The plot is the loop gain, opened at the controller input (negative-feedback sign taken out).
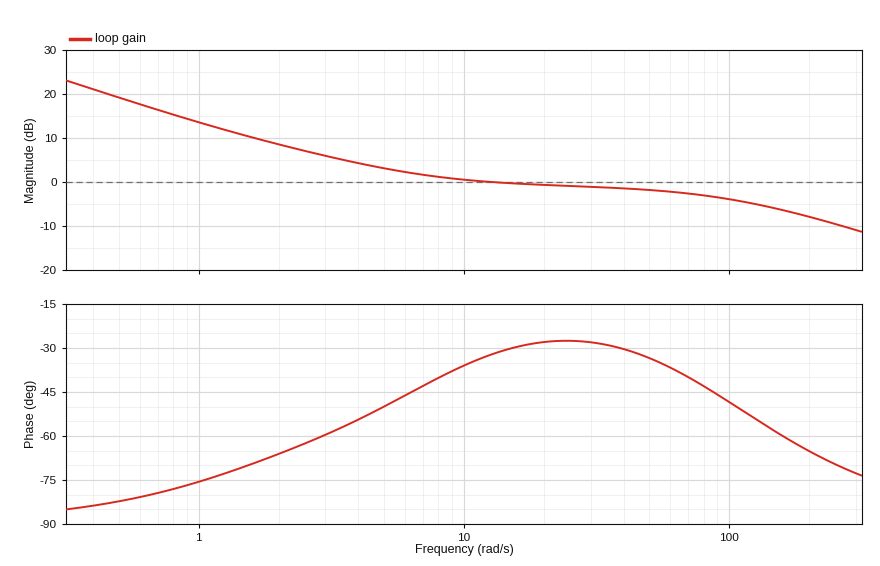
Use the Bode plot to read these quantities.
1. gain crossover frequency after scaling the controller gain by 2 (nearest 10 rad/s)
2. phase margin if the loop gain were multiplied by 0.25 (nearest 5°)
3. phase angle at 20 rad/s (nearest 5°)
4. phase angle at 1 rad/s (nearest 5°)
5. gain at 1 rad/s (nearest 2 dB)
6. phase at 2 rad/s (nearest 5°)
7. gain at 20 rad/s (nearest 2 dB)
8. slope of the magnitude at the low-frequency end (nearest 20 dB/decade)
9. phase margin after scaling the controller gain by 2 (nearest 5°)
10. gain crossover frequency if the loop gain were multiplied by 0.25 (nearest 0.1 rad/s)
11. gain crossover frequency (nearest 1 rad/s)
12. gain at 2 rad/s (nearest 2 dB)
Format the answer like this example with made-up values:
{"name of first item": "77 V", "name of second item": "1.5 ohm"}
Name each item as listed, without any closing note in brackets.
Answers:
{"gain crossover frequency after scaling the controller gain by 2": "150 rad/s", "phase margin if the loop gain were multiplied by 0.25": "105°", "phase angle at 20 rad/s": "-30°", "phase angle at 1 rad/s": "-75°", "gain at 1 rad/s": "14 dB", "phase at 2 rad/s": "-65°", "gain at 20 rad/s": "0 dB", "slope of the magnitude at the low-frequency end": "-20 dB/decade", "phase margin after scaling the controller gain by 2": "120°", "gain crossover frequency if the loop gain were multiplied by 0.25": "1.2 rad/s", "gain crossover frequency": "13 rad/s", "gain at 2 rad/s": "8 dB"}
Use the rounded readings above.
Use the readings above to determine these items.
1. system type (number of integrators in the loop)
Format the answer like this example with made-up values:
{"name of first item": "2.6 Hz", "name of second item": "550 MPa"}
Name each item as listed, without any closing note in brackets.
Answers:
{"system type": "1"}
